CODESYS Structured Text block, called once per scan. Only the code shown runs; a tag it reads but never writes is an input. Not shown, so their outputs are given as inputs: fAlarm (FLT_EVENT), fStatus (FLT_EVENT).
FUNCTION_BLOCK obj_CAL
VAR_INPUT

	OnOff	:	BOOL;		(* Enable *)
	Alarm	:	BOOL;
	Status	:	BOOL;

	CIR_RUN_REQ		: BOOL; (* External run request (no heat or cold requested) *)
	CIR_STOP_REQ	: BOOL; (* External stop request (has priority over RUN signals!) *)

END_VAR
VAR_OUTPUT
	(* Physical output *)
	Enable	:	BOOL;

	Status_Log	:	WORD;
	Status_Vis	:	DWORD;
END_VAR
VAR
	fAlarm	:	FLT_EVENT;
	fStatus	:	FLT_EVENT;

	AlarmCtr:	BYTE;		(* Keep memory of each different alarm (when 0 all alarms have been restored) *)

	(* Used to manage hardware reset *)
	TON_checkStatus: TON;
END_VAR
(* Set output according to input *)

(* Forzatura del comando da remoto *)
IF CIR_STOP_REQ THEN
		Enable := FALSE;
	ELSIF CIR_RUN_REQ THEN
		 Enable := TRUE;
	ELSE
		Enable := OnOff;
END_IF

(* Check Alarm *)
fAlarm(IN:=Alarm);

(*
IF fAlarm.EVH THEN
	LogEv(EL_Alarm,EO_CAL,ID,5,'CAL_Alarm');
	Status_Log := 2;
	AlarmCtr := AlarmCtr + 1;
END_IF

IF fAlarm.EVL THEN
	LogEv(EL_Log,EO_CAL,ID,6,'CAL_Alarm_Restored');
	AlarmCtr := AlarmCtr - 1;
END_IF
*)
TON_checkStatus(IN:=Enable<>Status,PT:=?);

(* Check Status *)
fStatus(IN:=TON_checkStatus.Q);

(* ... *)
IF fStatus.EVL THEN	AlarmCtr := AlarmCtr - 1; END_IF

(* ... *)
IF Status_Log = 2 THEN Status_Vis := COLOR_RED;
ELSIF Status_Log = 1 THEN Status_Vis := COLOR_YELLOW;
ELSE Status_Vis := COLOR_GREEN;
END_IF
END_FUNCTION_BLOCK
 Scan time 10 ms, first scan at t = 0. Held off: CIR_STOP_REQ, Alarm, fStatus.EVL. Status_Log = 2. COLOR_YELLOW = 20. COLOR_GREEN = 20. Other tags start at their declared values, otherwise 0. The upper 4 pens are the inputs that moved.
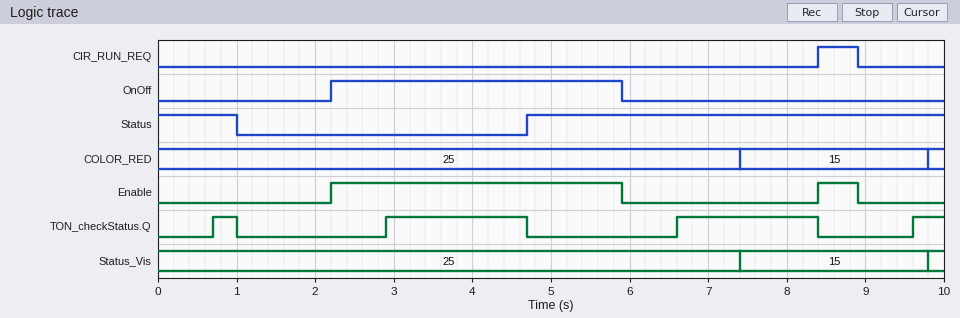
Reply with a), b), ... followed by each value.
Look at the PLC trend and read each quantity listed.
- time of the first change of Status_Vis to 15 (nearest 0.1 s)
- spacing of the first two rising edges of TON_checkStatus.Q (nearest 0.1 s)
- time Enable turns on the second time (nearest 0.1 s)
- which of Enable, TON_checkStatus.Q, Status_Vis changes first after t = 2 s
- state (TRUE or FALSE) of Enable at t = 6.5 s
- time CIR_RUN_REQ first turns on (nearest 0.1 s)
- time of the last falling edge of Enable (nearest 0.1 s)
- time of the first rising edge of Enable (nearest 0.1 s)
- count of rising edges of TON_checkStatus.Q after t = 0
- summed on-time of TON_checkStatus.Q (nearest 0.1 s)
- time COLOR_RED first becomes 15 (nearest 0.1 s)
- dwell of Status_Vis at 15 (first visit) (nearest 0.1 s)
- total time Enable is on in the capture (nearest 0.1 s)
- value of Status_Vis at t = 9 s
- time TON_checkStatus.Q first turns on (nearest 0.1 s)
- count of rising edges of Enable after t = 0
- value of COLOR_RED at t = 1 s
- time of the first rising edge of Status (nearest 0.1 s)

a) 7.4 s
b) 2.2 s
c) 8.4 s
d) Enable
e) FALSE
f) 8.4 s
g) 8.9 s
h) 2.2 s
i) 4
j) 4.3 s
k) 7.4 s
l) 2.4 s
m) 4.2 s
n) 15
o) 0.7 s
p) 2
q) 25
r) 4.7 s
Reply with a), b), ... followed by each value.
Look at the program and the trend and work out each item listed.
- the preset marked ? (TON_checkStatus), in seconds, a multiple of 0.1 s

a) 0.7 s
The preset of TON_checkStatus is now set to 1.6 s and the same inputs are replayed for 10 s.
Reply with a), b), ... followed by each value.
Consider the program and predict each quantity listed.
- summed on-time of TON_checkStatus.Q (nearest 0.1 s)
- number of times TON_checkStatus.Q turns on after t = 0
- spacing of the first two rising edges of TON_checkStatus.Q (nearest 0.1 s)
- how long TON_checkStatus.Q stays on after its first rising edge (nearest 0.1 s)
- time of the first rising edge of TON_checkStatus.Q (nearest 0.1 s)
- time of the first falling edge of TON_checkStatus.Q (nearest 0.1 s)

a) 1.8 s
b) 2
c) 3.7 s
d) 0.9 s
e) 3.8 s
f) 4.7 s
